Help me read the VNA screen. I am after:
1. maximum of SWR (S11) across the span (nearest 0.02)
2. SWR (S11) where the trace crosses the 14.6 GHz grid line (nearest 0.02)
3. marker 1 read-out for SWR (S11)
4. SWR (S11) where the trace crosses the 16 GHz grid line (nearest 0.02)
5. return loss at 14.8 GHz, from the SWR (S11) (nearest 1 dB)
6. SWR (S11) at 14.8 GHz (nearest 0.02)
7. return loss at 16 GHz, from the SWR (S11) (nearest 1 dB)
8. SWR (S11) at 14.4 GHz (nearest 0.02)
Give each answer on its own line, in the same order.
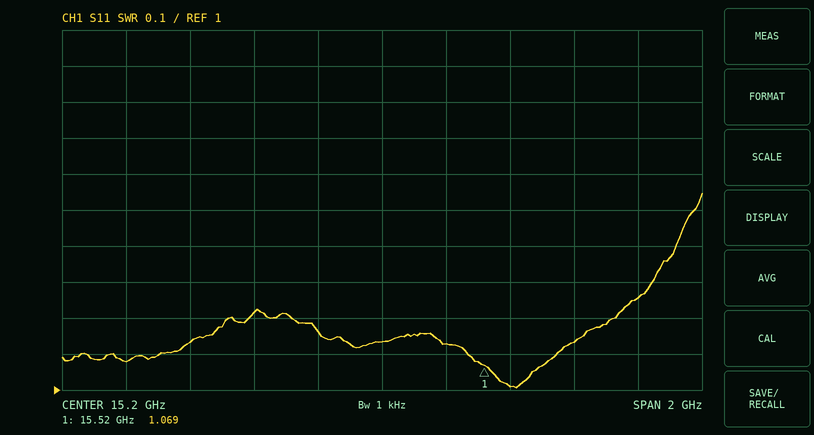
1.54
1.14
1.069
1.26
20 dB
1.22
19 dB
1.08
